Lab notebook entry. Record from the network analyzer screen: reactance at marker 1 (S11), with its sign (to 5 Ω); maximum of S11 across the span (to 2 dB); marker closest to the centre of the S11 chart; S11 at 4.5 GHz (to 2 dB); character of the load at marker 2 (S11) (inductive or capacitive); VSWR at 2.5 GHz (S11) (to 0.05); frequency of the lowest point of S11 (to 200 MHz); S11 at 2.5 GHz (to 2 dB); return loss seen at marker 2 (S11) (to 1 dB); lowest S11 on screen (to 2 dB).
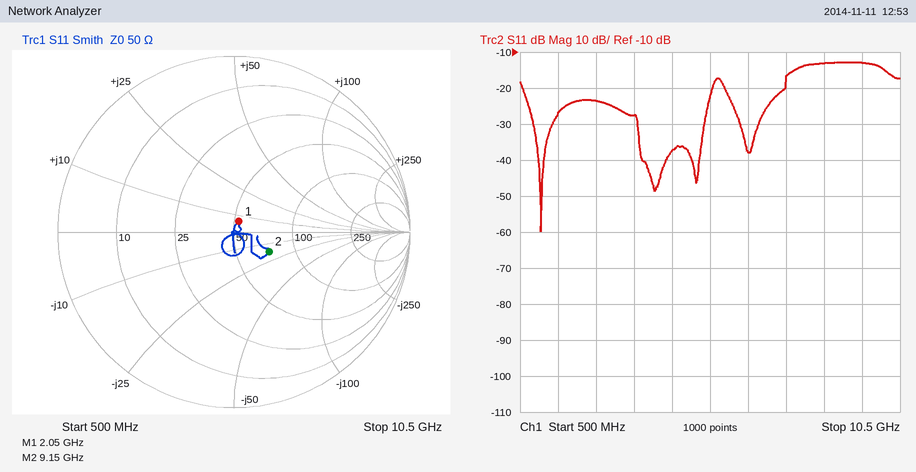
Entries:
+5 Ω
-12 dB
marker 1
-38 dB
capacitive
1.15
1.0 GHz
-24 dB
13 dB
-60 dB
